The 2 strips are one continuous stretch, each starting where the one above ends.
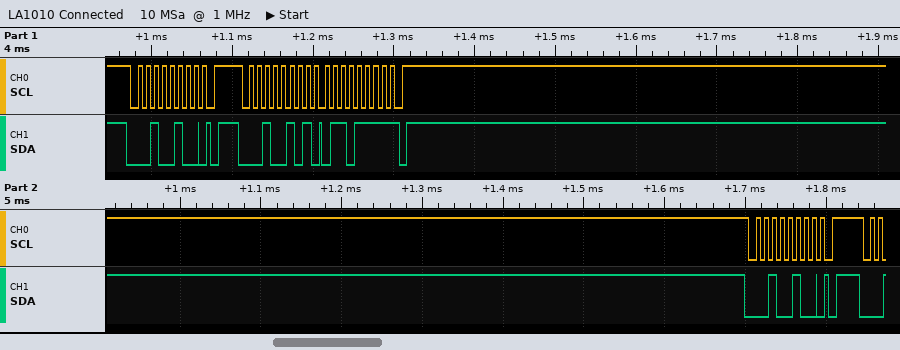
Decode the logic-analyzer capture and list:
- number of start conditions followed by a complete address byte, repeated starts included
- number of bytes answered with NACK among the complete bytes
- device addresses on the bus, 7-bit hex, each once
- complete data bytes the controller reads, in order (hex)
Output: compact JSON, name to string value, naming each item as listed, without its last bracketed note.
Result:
{"number of start conditions followed by a complete address byte, repeated starts included": "3", "number of bytes answered with NACK among the complete bytes": "1", "device addresses on the bus, 7-bit hex, each once": "0x12", "complete data bytes the controller reads, in order": "6F"}
